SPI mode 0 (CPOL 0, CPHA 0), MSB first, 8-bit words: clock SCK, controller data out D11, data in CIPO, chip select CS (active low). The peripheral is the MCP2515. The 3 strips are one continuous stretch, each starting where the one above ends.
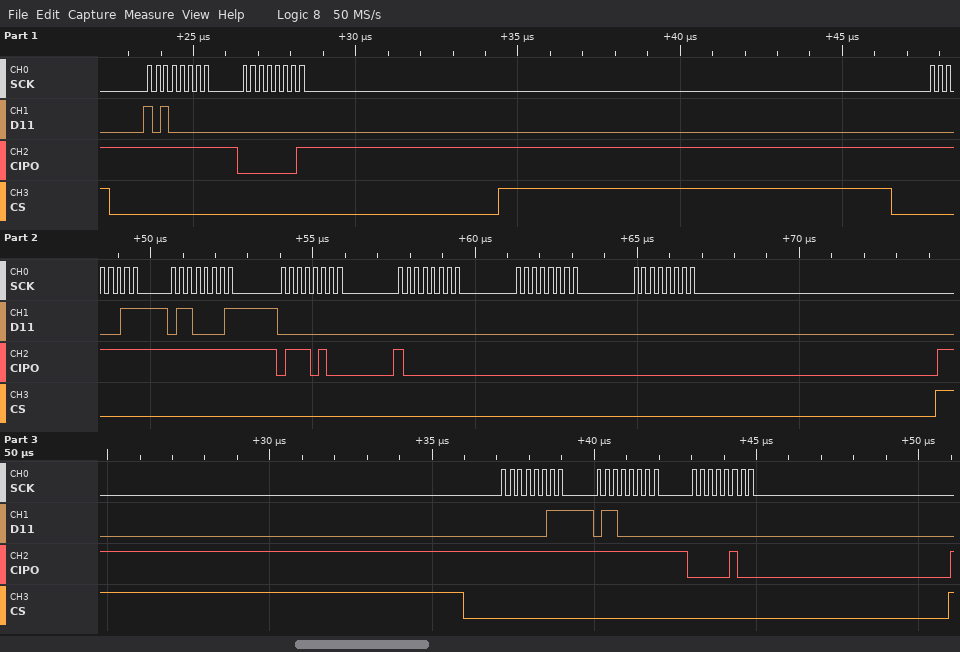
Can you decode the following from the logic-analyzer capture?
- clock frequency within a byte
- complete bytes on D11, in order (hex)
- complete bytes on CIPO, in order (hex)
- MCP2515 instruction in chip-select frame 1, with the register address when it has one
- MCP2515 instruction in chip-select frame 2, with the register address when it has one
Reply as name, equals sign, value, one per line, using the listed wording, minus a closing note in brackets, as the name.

clock frequency within a byte = 4 MHz
complete bytes on D11, in order = A0 00 03 61 00 00 00 00 03 60 00
complete bytes on CIPO, in order = FF 01 FF FF 74 80 00 00 FF FF 04
MCP2515 instruction in chip-select frame 1, with the register address when it has one = READ STATUS
MCP2515 instruction in chip-select frame 2, with the register address when it has one = READ 0x61
